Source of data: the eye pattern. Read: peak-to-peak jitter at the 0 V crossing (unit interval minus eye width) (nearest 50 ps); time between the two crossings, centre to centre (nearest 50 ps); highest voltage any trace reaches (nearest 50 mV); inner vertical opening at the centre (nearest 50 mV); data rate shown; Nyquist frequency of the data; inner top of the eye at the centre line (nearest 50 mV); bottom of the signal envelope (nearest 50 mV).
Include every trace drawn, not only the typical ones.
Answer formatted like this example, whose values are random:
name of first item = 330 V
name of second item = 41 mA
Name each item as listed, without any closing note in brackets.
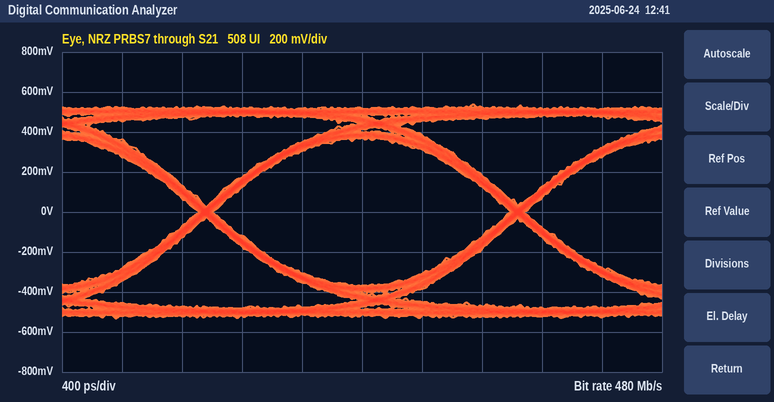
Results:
peak-to-peak jitter at the 0 V crossing (unit interval minus eye width) = 100 ps
time between the two crossings, centre to centre = 2.10 ns
highest voltage any trace reaches = 550 mV
inner vertical opening at the centre = 750 mV
data rate shown = 480 Mb/s
Nyquist frequency of the data = 240 MHz
inner top of the eye at the centre line = 350 mV
bottom of the signal envelope = -550 mV
